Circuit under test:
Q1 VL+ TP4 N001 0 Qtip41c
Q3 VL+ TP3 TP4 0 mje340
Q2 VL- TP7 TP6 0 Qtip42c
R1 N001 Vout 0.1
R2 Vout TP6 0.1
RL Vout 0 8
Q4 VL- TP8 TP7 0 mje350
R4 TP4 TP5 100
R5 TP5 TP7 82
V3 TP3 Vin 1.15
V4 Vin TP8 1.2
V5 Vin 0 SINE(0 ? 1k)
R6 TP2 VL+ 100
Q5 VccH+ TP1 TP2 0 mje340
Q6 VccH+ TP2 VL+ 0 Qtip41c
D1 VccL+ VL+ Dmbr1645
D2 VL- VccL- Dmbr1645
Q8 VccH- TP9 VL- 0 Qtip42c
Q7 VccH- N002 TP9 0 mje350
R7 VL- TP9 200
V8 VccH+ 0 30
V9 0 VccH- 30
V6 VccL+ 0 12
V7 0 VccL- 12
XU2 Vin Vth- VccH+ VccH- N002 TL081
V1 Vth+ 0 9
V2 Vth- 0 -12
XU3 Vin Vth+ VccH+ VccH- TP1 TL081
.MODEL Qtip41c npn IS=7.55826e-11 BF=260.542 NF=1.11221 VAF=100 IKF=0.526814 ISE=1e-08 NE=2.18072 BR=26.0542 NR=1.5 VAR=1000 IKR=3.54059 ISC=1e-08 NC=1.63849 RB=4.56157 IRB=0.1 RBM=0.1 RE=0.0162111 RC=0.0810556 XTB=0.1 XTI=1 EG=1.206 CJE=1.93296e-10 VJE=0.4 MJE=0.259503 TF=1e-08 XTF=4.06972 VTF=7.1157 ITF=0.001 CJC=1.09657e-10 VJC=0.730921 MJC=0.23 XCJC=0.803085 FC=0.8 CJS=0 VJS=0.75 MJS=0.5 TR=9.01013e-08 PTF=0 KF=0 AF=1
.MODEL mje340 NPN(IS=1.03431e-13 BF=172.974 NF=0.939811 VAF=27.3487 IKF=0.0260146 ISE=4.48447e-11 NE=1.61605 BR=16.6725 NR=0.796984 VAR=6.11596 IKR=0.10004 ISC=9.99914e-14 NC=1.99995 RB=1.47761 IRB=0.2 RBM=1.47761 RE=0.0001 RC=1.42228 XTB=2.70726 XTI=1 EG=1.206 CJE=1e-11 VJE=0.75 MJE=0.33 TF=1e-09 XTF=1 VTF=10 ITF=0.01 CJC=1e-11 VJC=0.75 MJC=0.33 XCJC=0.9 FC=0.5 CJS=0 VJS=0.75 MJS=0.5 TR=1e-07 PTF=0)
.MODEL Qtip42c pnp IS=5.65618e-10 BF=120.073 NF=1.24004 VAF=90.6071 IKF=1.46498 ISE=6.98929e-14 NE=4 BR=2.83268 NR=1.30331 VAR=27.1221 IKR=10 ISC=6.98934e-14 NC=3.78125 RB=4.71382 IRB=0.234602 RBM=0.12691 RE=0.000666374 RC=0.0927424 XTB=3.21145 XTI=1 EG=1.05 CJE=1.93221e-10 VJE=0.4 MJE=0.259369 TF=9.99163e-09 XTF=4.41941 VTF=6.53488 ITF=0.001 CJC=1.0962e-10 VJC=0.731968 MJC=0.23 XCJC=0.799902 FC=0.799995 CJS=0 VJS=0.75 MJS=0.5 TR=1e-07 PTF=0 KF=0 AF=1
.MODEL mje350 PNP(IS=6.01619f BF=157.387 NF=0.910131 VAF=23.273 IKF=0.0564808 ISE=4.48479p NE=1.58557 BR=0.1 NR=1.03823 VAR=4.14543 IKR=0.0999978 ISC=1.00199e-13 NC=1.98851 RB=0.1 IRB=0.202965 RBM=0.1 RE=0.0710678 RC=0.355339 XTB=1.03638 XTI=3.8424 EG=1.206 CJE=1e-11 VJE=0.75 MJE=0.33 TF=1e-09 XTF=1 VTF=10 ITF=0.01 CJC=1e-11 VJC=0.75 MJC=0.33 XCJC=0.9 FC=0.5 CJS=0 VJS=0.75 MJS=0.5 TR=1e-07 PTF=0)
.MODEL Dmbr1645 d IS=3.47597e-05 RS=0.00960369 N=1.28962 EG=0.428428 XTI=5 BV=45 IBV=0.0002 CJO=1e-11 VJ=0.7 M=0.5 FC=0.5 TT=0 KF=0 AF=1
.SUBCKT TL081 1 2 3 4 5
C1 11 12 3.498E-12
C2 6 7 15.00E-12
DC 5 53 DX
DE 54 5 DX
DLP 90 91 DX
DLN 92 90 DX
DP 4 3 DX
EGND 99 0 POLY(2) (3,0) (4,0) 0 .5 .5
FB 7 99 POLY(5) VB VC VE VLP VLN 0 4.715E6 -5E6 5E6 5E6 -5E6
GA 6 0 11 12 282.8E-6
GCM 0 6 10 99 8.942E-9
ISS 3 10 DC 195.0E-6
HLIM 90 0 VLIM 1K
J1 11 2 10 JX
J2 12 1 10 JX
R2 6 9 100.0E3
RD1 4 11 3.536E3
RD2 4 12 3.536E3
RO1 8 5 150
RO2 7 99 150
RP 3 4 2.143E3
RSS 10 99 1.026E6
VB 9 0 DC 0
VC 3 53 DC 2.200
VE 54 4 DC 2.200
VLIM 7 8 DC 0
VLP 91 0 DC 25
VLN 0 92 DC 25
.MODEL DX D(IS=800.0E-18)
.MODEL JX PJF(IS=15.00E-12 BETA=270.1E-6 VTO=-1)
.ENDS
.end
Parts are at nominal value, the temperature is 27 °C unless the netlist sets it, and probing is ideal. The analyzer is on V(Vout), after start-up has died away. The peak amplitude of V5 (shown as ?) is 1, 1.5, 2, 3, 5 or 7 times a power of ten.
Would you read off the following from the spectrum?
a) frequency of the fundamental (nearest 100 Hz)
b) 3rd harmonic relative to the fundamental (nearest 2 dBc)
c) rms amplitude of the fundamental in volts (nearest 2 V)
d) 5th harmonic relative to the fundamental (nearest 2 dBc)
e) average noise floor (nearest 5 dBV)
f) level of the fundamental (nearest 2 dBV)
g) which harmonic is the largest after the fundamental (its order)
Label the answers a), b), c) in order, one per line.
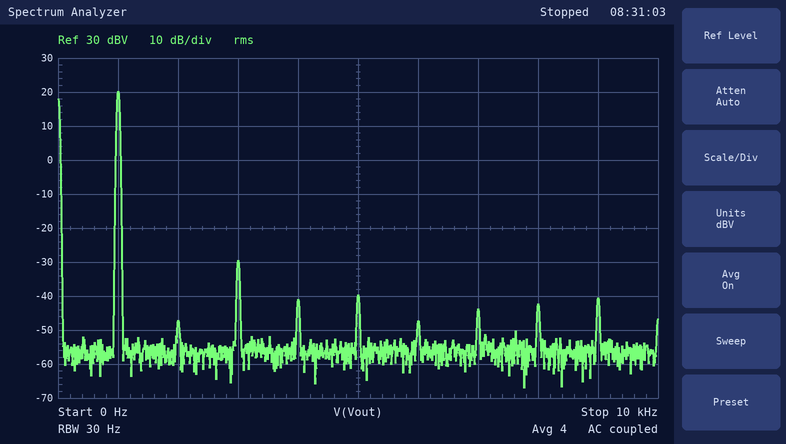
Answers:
a) 1.0 kHz
b) -50 dBc
c) 10 V
d) -60 dBc
e) -55 dBV
f) 20 dBV
g) 3
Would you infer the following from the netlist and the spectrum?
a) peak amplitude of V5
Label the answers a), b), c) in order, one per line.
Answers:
a) 15 V
